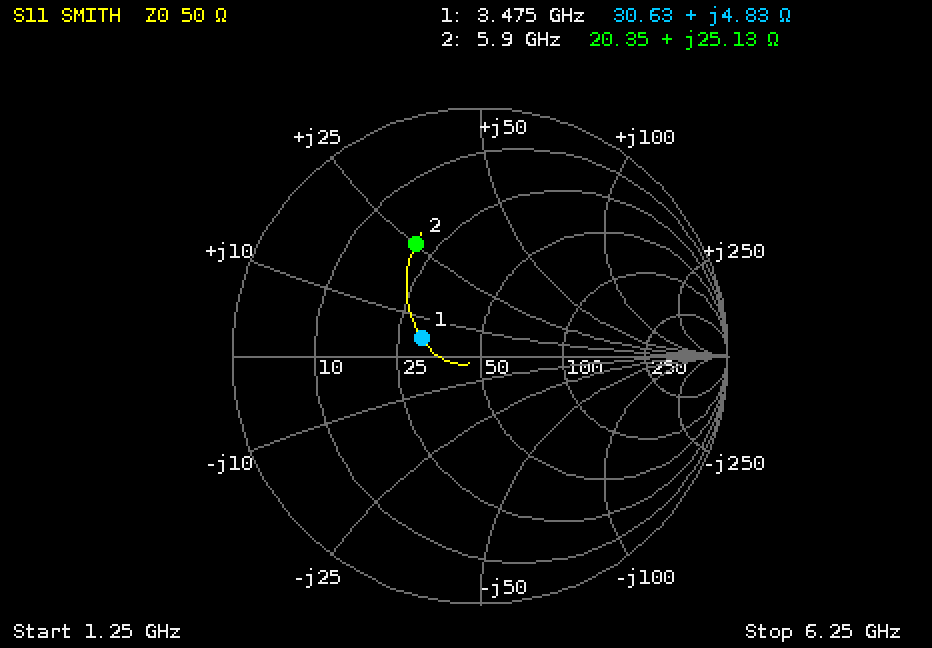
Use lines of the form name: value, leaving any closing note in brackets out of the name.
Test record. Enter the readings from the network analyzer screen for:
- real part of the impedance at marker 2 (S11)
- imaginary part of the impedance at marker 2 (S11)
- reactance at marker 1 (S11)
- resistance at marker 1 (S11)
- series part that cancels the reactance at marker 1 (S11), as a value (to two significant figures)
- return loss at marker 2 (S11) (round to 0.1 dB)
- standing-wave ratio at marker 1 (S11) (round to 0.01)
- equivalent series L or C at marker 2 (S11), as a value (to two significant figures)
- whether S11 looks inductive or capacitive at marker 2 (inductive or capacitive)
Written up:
real part of the impedance at marker 2: 20.35 Ω
imaginary part of the impedance at marker 2: +25.13 Ω
reactance at marker 1: +4.83 Ω
resistance at marker 1: 30.63 Ω
series part that cancels the reactance at marker 1 (S11), as a value: 9.5 pF
return loss at marker 2 (S11): 5.7 dB
standing-wave ratio at marker 1 (S11): 1.66
equivalent series L or C at marker 2 (S11), as a value: 680 pH
whether S11 looks inductive or capacitive at marker 2: inductive
